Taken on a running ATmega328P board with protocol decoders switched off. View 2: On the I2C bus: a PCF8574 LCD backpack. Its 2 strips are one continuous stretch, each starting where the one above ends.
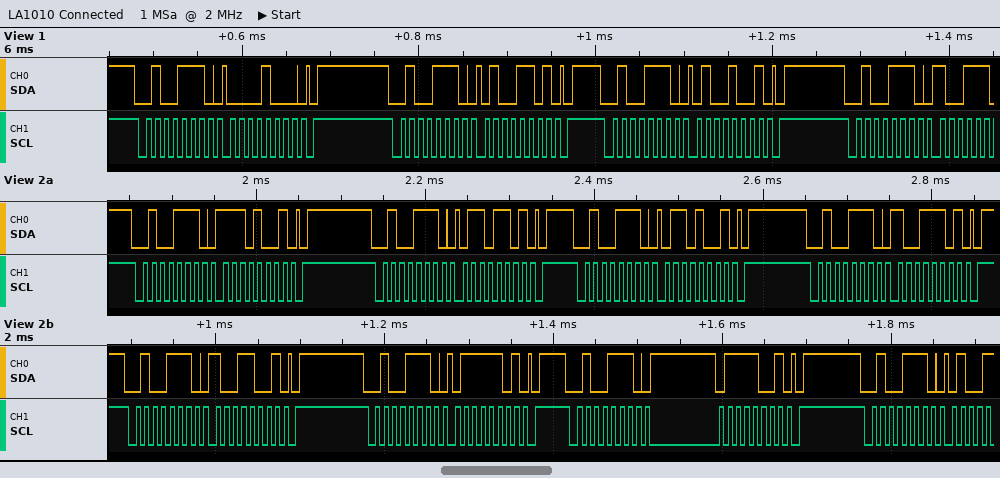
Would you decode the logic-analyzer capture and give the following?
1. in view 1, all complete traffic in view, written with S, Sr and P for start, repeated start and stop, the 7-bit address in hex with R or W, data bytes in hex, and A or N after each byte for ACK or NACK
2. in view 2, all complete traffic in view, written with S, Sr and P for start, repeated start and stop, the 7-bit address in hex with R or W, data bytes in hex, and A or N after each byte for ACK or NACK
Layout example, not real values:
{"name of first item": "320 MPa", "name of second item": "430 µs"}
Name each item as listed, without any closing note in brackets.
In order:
{"in view 1, all complete traffic in view, written with S, Sr and P for start, repeated start and stop, the 7-bit address in hex with R or W, data bytes in hex, and A or N after each byte for ACK or NACK": "S 27W A 08 A P S 27W A 4D A P S 27W A 49 A P S 27W A", "in view 2, all complete traffic in view, written with S, Sr and P for start, repeated start and stop, the 7-bit address in hex with R or W, data bytes in hex, and A or N after each byte for ACK or NACK": "S 27W A E9 A P S 27W A 6D A P S 27W A 69 A P S 27W A 9D A P S 27W A 99 A P S 27W A 7D A P S 27W A 79 A P S 27W A"}
